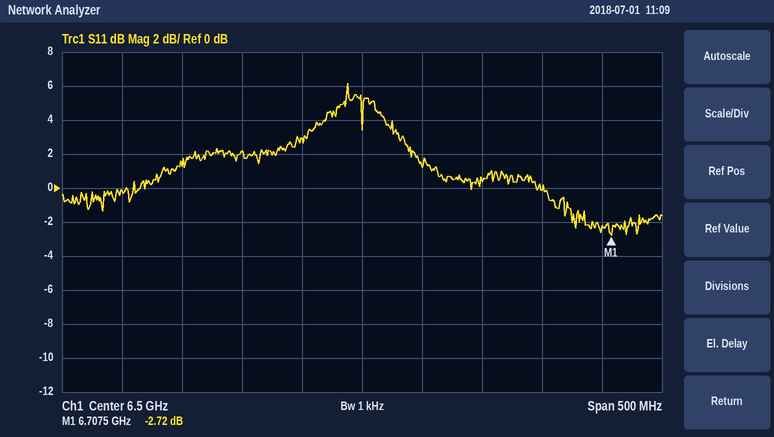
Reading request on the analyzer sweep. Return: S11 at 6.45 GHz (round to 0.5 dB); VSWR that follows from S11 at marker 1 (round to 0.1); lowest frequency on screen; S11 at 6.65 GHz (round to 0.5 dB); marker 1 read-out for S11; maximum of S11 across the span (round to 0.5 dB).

3.0 dB
6.4
6.25 GHz
0.0 dB
-2.72 dB
6.0 dB
